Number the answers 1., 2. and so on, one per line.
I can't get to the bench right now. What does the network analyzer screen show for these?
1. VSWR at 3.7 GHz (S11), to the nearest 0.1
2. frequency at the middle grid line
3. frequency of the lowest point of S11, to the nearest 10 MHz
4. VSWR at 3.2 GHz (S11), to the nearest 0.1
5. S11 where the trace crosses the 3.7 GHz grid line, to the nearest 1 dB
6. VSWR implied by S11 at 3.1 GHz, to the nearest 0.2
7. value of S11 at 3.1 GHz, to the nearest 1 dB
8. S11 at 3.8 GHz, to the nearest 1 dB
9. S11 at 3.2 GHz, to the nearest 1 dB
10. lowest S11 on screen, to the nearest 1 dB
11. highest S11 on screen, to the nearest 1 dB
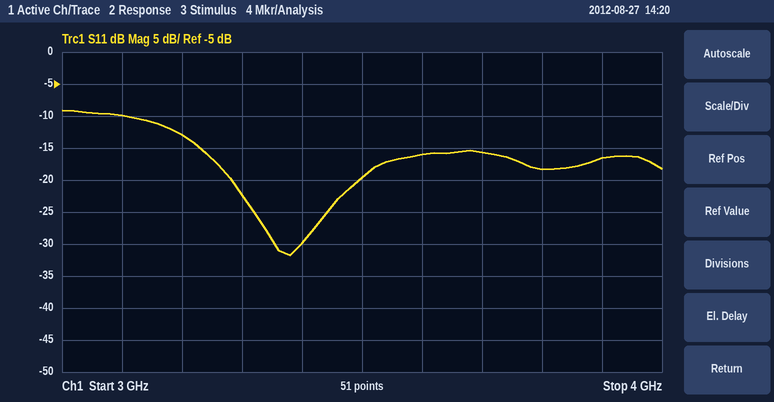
1. 1.4
2. 3.5 GHz
3. 3.38 GHz
4. 1.6
5. -16 dB
6. 2.0
7. -10 dB
8. -18 dB
9. -13 dB
10. -32 dB
11. -9 dB
